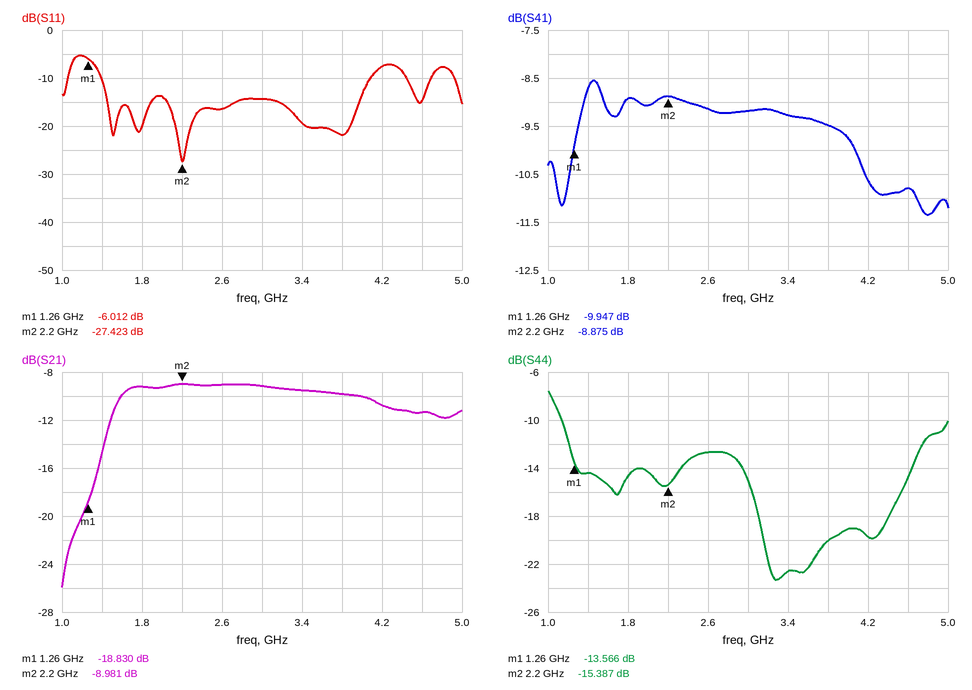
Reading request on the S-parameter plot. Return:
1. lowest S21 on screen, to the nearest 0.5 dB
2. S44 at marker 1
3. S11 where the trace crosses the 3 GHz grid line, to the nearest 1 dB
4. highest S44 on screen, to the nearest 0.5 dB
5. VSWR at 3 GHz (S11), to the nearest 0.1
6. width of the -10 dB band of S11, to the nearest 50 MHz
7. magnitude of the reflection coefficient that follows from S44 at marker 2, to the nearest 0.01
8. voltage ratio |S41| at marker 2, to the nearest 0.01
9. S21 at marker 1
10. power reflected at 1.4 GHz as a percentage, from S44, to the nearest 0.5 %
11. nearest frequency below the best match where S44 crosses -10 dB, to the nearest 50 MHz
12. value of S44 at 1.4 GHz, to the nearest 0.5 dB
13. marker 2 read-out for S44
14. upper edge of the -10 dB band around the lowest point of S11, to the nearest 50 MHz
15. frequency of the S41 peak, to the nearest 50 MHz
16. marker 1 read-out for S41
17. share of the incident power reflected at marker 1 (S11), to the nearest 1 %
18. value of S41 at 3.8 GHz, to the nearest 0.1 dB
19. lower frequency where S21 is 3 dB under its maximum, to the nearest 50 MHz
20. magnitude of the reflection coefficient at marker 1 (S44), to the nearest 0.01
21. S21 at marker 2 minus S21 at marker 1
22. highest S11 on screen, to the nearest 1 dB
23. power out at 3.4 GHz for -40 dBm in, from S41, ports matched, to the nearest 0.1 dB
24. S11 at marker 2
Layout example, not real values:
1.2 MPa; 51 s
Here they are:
-26.0 dB; -13.566 dB; -14 dB; -7.5 dB; 1.5; 2.70 GHz; 0.17; 0.36; -18.830 dB; 3.5 %; 1.15 GHz; -14.5 dB; -15.387 dB; 4.10 GHz; 1.45 GHz; -9.947 dB; 25 %; -9.5 dB; 1.50 GHz; 0.21; 9.849 dB; -5 dB; -49.3 dBm; -27.423 dB
